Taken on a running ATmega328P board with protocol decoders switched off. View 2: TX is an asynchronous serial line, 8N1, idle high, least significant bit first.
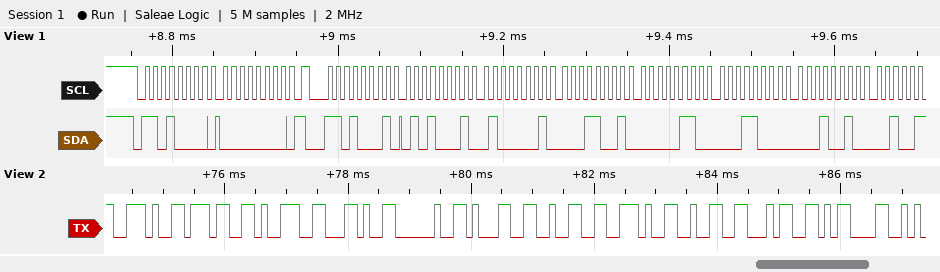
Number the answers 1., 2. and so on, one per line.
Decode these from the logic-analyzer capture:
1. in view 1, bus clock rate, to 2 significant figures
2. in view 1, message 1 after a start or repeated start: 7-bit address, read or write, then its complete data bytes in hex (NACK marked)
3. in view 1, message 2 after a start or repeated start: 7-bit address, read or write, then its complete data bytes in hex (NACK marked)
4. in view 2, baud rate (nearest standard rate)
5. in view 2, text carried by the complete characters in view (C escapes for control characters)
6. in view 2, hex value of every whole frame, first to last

1. 100 kHz
2. 0x68 write: 00
3. 0x68 read: 51 41 19 06 18 12
4. 9600 baud
5. ".79, 12.24\r"
6. 2E 37 39 2C 20 31 32 2E 32 34 0D
